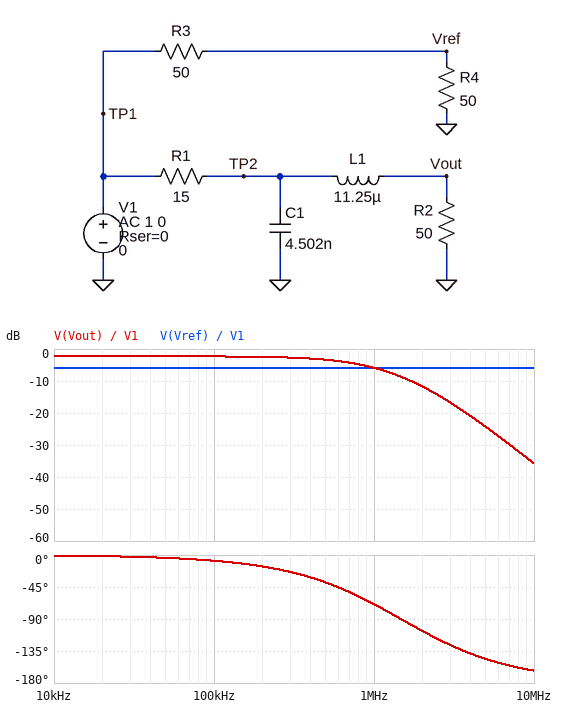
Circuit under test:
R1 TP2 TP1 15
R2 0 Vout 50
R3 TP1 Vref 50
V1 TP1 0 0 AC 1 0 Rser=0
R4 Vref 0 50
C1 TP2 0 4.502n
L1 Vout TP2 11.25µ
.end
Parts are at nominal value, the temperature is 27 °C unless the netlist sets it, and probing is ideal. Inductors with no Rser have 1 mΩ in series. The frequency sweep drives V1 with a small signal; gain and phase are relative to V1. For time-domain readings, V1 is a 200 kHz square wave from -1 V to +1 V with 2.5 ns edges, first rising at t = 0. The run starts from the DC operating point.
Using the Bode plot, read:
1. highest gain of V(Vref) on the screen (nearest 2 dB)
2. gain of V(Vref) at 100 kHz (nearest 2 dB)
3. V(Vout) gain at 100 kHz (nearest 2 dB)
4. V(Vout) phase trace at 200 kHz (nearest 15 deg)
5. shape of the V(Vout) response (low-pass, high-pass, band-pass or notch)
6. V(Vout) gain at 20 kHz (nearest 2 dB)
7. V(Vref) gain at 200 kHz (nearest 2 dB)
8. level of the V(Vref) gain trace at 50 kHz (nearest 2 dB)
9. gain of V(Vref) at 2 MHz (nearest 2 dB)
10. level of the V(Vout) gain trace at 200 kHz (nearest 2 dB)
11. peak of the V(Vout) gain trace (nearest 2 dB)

-6 dB
-6 dB
-2 dB
-15 deg
low-pass
-2 dB
-6 dB
-6 dB
-6 dB
-2 dB
-2 dB
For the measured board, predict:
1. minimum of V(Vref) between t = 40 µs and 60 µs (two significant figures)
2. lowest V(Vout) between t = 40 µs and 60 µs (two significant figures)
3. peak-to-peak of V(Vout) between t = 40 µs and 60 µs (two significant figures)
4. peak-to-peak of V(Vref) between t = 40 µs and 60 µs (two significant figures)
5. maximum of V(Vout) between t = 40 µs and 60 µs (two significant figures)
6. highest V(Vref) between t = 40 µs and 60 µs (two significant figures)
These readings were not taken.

-500 mV
-770 mV
1.5 V
1.0 V
770 mV
500 mV
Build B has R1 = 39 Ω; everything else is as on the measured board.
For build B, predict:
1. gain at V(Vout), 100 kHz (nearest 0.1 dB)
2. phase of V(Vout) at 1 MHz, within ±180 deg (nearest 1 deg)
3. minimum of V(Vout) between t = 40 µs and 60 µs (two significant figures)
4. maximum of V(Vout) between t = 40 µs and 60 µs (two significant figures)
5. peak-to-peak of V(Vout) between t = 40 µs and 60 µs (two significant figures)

-5.0 dB
-85 deg
-590 mV
590 mV
1.2 V
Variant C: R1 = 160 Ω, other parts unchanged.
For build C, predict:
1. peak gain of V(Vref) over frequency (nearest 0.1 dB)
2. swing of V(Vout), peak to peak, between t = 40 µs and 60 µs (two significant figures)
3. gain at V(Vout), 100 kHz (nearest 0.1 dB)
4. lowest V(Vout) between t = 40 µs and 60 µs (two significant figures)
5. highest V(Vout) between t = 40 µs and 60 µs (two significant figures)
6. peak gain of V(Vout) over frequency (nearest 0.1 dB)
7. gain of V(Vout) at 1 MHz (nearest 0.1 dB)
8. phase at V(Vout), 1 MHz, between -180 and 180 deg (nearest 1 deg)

-6.0 dB
580 mV
-12.4 dB
-290 mV
290 mV
-11.9 dB
-16.0 dB
-110 deg
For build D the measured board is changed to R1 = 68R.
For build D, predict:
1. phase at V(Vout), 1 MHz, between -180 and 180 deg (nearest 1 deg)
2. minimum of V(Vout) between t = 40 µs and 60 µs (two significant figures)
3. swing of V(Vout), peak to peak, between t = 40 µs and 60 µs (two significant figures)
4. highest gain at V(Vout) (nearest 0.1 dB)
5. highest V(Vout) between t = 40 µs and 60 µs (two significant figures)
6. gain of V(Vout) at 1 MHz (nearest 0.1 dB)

-96 deg
-480 mV
960 mV
-7.4 dB
480 mV
-10.5 dB
